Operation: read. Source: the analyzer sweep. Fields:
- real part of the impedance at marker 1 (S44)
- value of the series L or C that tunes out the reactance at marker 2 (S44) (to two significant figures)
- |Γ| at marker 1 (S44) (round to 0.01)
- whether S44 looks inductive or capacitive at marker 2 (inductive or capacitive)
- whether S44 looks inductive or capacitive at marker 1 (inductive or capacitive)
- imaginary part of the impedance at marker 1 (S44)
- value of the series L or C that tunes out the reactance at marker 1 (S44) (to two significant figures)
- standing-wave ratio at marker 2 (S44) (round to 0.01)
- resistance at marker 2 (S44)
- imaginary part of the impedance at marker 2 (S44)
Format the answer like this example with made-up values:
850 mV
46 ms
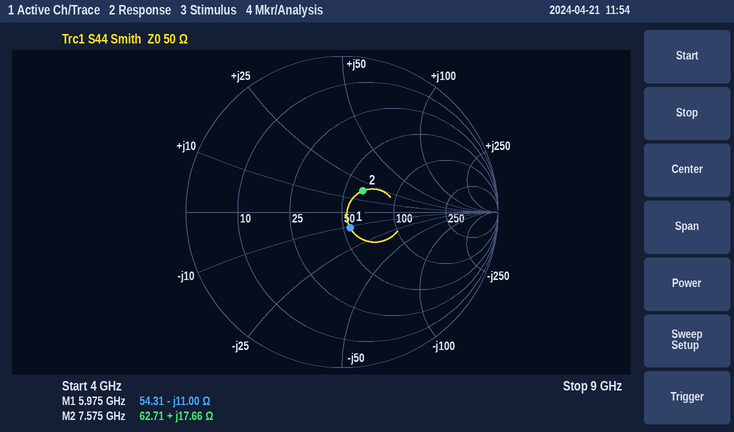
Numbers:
54.31 Ω
1.2 pF
0.11
inductive
capacitive
-11.00 Ω
290 pH
1.47
62.71 Ω
+17.66 Ω
